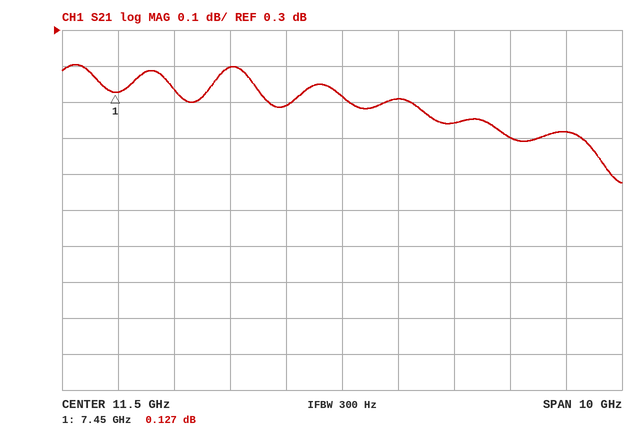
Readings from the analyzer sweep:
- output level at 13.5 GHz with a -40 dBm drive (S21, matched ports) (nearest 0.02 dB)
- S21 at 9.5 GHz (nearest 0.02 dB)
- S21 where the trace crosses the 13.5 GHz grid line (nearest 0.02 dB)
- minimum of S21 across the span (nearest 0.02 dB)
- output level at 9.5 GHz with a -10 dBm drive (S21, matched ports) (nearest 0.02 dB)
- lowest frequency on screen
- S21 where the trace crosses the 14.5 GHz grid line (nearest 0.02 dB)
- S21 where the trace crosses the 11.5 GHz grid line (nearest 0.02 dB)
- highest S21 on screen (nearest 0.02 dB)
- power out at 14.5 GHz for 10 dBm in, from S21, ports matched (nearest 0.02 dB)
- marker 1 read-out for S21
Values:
-39.96 dBm
0.20 dB
0.04 dB
-0.12 dB
-9.80 dBm
6.5 GHz
0.00 dB
0.12 dB
0.20 dB
10.00 dBm
0.127 dB
